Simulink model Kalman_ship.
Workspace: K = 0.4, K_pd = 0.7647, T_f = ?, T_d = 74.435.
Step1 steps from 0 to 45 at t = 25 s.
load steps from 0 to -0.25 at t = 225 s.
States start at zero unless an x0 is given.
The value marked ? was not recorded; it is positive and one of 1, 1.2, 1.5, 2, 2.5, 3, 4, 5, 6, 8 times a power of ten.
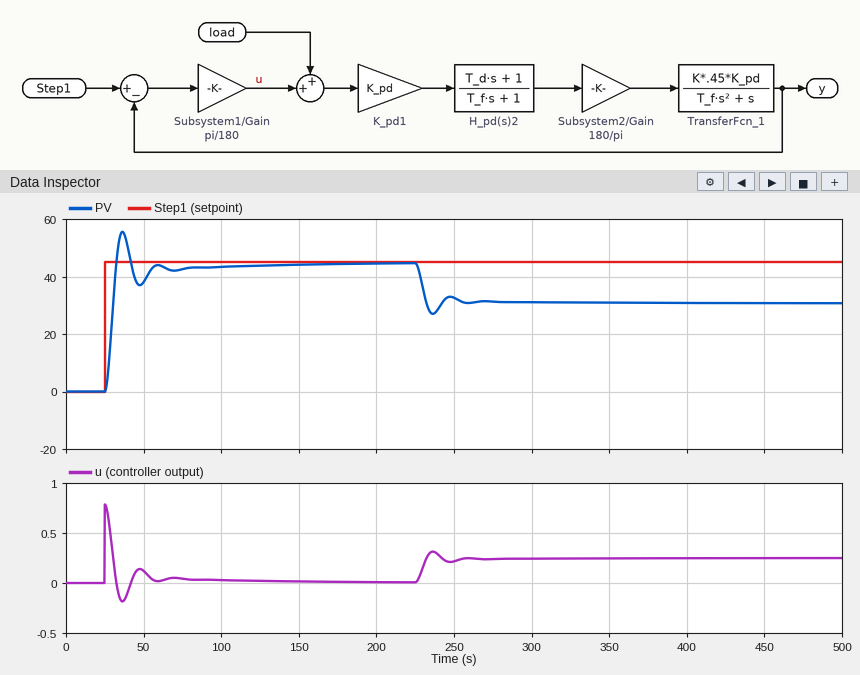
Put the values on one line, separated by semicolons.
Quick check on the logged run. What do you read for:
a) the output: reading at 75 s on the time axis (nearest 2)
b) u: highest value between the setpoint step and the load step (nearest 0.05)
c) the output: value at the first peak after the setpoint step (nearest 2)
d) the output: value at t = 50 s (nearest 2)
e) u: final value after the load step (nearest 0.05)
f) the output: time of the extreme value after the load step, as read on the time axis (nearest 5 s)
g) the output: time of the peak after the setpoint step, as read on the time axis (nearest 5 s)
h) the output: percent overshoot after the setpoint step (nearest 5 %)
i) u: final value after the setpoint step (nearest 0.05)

42; 0.80; 56; 38; 0.25; 235 s; 35 s; 25 %; 0.00
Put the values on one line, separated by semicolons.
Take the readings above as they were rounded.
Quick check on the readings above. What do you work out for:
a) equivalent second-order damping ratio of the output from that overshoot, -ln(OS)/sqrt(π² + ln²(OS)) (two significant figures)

0.40
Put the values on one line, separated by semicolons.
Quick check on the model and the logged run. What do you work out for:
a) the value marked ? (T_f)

10
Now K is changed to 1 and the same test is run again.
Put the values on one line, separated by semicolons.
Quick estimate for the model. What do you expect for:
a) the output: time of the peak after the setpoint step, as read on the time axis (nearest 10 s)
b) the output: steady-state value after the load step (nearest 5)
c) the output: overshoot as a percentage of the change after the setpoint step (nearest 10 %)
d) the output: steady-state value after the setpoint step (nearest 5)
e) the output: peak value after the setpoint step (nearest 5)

30 s; 30; 50 %; 45; 65
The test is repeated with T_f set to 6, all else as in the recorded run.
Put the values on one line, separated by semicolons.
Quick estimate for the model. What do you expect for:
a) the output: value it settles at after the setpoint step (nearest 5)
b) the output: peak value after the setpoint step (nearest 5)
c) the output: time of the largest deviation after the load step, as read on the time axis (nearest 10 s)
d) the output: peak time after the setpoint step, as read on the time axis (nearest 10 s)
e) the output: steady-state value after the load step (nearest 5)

45; 55; 230 s; 30 s; 30
